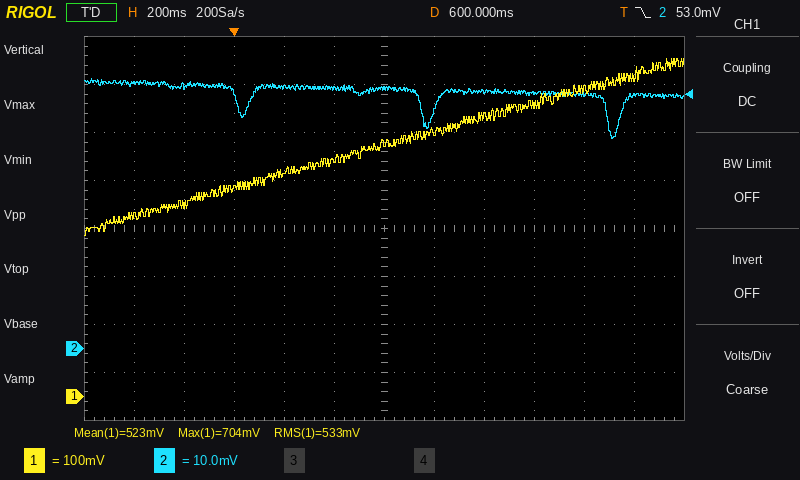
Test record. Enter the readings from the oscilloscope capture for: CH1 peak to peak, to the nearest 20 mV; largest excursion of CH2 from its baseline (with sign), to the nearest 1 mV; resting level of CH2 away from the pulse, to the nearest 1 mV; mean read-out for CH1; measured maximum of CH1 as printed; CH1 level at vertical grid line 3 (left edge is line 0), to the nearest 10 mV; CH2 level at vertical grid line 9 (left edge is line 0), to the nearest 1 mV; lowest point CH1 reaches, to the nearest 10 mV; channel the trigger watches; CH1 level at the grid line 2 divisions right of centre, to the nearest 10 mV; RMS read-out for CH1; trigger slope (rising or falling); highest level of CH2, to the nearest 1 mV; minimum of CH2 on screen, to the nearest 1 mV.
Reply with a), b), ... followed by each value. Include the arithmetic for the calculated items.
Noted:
a) 360 mV
b) 44 mV − (54 mV) = -10 mV
c) 54 mV
d) 523 mV
e) 704 mV
f) 430 mV
g) 53 mV
h) 340 mV
i) CH2
j) 580 mV
k) 533 mV
l) falling
m) 56 mV
n) 44 mV
